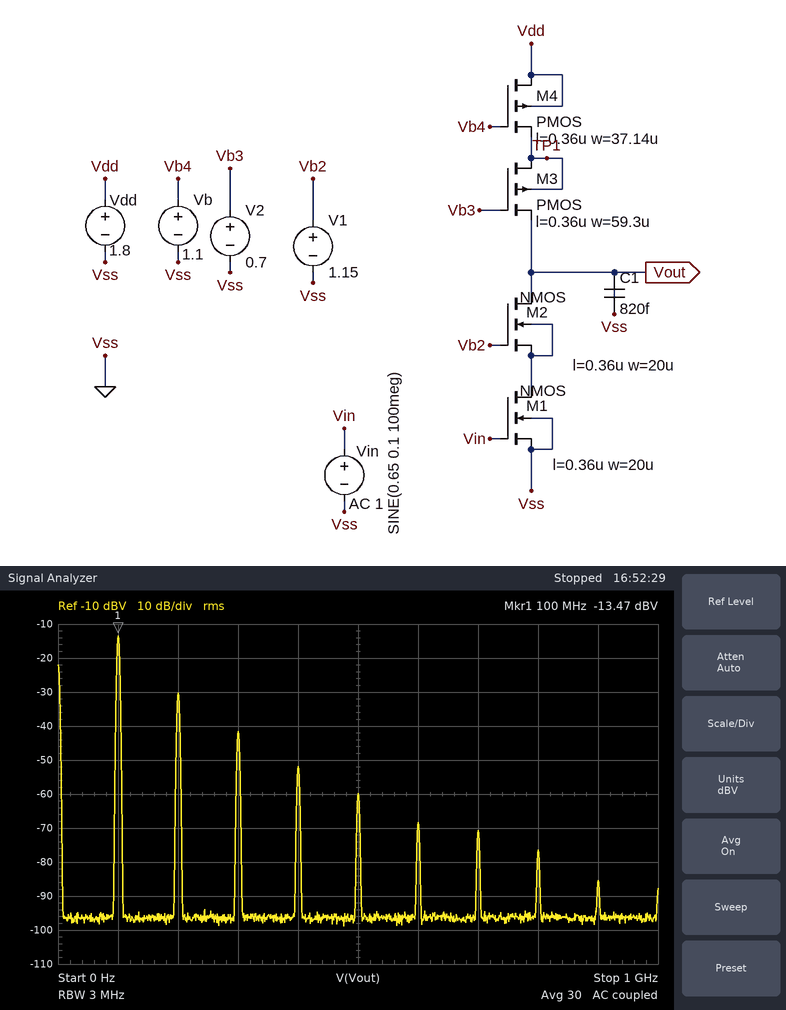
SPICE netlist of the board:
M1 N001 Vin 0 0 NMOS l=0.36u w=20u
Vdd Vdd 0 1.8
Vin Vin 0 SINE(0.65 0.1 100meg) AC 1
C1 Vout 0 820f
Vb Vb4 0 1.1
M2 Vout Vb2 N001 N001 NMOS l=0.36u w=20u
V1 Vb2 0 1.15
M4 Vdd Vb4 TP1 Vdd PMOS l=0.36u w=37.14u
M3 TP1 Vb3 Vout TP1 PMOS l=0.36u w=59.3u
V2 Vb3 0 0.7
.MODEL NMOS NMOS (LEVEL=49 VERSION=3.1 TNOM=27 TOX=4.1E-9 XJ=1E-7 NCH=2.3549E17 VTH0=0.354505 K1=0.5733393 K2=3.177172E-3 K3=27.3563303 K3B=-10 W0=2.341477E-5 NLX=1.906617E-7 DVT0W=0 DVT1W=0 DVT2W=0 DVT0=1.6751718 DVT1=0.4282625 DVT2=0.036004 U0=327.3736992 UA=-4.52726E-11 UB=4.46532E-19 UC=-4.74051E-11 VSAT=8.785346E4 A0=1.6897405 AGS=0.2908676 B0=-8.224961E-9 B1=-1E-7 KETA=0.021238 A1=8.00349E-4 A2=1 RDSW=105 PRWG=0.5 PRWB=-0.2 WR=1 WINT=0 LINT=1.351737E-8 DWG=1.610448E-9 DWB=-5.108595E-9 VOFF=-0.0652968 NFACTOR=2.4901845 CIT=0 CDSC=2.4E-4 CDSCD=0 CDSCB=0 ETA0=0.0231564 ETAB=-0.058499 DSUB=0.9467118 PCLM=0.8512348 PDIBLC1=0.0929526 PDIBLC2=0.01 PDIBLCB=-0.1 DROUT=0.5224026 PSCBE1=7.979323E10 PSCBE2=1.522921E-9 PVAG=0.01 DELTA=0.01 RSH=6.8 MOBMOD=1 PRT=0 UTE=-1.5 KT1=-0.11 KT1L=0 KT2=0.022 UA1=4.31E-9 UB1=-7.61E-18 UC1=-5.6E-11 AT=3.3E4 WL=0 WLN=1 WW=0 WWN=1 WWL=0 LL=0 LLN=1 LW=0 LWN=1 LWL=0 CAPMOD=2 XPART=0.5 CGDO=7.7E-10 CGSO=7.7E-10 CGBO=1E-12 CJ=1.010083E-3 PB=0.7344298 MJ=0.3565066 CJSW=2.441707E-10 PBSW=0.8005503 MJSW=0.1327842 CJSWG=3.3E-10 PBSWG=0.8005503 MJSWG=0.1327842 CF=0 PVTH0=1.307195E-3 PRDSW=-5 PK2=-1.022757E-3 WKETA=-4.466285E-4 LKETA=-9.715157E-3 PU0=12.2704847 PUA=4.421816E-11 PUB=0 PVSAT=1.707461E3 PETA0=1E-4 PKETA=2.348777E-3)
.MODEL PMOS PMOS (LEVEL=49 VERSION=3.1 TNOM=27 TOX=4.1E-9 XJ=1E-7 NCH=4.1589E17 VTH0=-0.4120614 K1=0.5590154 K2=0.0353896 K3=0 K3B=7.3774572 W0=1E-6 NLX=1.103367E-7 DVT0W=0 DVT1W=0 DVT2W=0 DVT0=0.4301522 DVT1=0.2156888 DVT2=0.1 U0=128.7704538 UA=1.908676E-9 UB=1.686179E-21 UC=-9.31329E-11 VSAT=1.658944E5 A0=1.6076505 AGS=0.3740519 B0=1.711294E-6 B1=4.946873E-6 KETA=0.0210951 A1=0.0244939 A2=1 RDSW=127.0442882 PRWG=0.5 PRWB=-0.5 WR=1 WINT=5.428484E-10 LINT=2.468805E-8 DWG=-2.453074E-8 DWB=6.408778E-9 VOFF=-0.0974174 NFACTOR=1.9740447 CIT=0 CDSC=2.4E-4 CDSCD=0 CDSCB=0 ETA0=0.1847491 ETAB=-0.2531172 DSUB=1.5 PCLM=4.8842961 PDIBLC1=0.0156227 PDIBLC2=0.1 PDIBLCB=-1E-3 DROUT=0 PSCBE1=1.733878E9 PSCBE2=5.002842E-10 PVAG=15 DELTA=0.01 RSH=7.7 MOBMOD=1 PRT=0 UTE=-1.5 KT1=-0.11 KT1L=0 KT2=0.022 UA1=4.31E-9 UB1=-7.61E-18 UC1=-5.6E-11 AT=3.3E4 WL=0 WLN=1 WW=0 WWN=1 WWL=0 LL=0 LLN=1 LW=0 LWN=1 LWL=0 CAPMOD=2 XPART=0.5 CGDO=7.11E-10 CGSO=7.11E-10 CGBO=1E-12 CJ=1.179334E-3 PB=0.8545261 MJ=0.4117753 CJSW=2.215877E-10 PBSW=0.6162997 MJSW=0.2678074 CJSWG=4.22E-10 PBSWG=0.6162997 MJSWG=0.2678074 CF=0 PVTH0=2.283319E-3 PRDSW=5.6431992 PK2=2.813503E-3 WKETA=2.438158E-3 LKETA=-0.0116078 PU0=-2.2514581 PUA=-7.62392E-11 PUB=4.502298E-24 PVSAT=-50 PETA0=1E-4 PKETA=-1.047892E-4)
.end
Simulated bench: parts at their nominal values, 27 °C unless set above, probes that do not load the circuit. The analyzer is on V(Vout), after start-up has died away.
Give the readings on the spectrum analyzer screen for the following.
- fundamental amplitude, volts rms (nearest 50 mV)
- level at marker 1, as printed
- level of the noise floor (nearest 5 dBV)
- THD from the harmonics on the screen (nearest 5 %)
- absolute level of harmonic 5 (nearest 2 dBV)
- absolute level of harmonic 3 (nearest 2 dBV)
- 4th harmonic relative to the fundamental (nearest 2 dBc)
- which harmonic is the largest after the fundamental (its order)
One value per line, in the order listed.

200 mV
-13.47 dBV
-95 dBV
15 %
-60 dBV
-42 dBV
-38 dBc
2
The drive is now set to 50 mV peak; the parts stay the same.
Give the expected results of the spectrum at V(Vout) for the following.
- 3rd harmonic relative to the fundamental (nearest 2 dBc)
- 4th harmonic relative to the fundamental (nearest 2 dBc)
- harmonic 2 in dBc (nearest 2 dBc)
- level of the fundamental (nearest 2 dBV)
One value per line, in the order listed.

-50 dBc
-58 dBc
-26 dBc
-18 dBV
